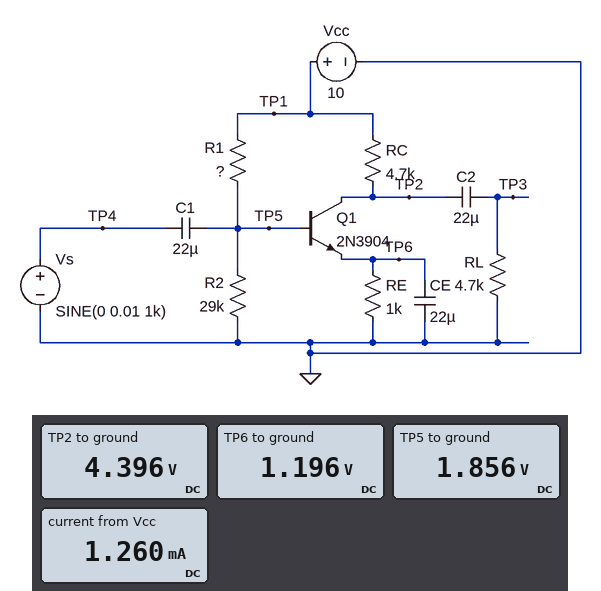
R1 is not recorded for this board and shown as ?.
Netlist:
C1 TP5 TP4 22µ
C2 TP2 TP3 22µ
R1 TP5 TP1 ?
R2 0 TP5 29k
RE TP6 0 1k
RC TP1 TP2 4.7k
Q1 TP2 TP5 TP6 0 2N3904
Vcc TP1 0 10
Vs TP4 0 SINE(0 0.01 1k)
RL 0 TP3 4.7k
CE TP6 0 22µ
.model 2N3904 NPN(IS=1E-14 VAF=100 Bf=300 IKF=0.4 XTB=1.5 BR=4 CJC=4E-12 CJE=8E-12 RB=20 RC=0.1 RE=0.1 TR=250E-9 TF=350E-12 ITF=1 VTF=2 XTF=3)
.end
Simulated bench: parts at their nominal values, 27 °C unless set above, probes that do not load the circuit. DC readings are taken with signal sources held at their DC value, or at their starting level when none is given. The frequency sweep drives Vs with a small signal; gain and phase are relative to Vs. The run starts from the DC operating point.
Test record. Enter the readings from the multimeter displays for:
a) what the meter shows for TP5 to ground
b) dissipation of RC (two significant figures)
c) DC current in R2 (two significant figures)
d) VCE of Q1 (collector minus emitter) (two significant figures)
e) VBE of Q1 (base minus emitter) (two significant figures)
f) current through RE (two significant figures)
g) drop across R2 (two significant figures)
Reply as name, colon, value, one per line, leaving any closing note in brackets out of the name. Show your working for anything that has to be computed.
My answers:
what the meter shows for TP5 to ground: 1.856 V
dissipation of RC: (10 V - 4.396 V)^2 / 4.7 kΩ = 6.7 mW
DC current in R2: (1.856 V) / 29 kΩ = 64 µA
VCE of Q1 (collector minus emitter): 4.396 V - 1.196 V = 3.2 V
VBE of Q1 (base minus emitter): 1.856 V - 1.196 V = 660 mV
current through RE: (1.196 V) / 1 kΩ = 1.2 mA
drop across R2: 1.856 V = 1.9 V
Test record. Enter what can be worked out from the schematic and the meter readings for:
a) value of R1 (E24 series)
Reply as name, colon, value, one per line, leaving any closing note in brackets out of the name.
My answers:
value of R1: 120 kΩ
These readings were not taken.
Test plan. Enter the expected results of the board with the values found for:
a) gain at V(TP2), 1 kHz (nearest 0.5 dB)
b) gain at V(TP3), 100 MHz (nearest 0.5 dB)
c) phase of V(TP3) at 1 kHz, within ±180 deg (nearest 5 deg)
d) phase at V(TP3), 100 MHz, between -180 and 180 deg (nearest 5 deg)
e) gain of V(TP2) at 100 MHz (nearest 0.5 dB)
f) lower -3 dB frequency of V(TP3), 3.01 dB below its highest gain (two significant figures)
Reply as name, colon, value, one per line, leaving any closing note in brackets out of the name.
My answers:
gain at V(TP2), 1 kHz: 40.0 dB
gain at V(TP3), 100 MHz: 23.5 dB
phase of V(TP3) at 1 kHz, within ±180 deg: -160 deg
phase at V(TP3), 100 MHz, between -180 and 180 deg: 85 deg
gain of V(TP2) at 100 MHz: 23.5 dB
lower -3 dB frequency of V(TP3), 3.01 dB below its highest gain: 330 Hz
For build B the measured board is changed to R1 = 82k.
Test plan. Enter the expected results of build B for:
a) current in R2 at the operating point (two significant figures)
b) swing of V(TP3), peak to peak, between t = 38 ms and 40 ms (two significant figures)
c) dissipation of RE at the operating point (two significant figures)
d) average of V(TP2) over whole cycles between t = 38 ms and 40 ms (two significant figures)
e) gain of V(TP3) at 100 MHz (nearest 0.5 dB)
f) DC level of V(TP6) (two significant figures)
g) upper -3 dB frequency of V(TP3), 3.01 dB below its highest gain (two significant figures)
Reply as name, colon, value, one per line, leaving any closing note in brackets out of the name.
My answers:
current in R2 at the operating point: 83 µA
swing of V(TP3), peak to peak, between t = 38 ms and 40 ms: 1.3 V
dissipation of RE at the operating point: 3.0 mW
average of V(TP2) over whole cycles between t = 38 ms and 40 ms: 2.2 V
gain of V(TP3) at 100 MHz: -5.5 dB
DC level of V(TP6): 1.7 V
upper -3 dB frequency of V(TP3), 3.01 dB below its highest gain: 620 kHz
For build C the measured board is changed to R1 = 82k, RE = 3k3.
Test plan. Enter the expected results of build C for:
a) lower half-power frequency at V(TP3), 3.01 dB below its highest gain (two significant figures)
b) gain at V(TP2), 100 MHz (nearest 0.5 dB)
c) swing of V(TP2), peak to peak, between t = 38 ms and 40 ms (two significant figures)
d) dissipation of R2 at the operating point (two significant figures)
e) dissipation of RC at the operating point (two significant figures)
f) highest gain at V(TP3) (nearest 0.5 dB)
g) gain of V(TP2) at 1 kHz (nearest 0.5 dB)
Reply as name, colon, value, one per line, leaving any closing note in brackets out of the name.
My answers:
lower half-power frequency at V(TP3), 3.01 dB below its highest gain: 160 Hz
gain at V(TP2), 100 MHz: 21.0 dB
swing of V(TP2), peak to peak, between t = 38 ms and 40 ms: 1.0 V
dissipation of R2 at the operating point: 230 µW
dissipation of RC at the operating point: 1.6 mW
highest gain at V(TP3): 34.5 dB
gain of V(TP2) at 1 kHz: 34.0 dB
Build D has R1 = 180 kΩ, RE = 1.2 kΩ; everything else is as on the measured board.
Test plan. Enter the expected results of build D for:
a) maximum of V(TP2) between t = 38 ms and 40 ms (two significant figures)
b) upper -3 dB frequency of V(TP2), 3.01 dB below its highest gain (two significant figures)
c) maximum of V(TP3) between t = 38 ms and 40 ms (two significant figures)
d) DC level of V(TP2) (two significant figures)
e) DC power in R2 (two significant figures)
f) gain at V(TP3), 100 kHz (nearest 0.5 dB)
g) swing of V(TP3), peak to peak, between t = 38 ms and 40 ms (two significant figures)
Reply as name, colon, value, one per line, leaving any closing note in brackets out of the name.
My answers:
maximum of V(TP2) between t = 38 ms and 40 ms: 7.7 V
upper -3 dB frequency of V(TP2), 3.01 dB below its highest gain: 24 MHz
maximum of V(TP3) between t = 38 ms and 40 ms: 460 mV
DC level of V(TP2): 7.3 V
DC power in R2: 62 µW
gain at V(TP3), 100 kHz: 34.5 dB
swing of V(TP3), peak to peak, between t = 38 ms and 40 ms: 1.0 V
